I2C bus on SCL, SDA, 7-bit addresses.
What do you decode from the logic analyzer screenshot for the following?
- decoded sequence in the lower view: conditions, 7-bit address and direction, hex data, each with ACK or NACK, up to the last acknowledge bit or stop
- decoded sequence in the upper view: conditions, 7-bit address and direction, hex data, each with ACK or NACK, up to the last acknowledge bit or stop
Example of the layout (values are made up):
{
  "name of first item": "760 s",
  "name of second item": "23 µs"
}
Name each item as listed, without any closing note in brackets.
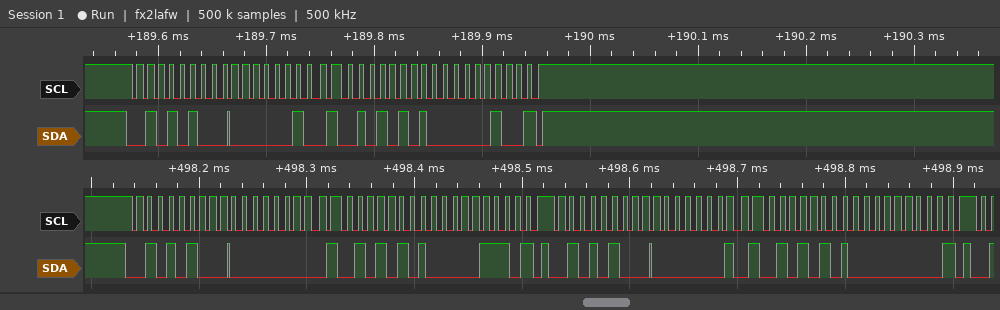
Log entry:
{
  "decoded sequence in the lower view: conditions, 7-bit address and direction, hex data, each with ACK or NACK, up to the last acknowledge bit or stop": "start, address 2A write ACK, 00 ACK, repeated start, address 2A read ACK, 0E NACK, stop, start, address 2A write ACK, 01 ACK, repeated start, address 2A read ACK, 00 NACK, stop",
  "decoded sequence in the upper view: conditions, 7-bit address and direction, hex data, each with ACK or NACK, up to the last acknowledge bit or stop": "start, address 2A write ACK, 02 ACK, repeated start, address 2A read ACK, 04 NACK, stop"
}
